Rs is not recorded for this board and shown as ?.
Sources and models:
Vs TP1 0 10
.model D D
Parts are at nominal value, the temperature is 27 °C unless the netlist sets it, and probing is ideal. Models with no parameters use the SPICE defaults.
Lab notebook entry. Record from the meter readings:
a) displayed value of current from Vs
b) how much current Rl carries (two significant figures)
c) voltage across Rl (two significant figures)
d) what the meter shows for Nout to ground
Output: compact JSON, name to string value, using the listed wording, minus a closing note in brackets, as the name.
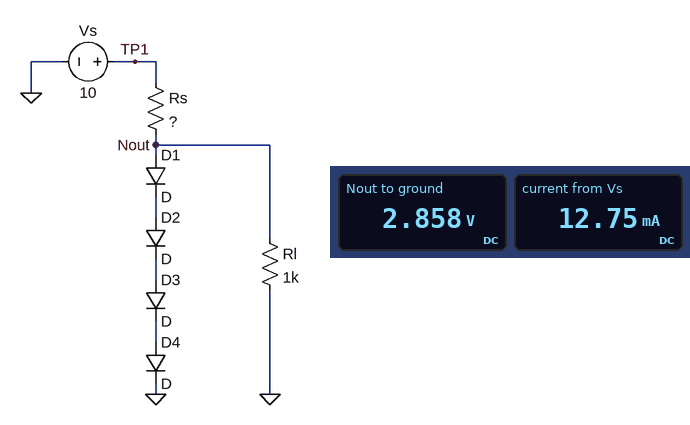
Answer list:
{"displayed value of current from Vs": "12.75 mA", "how much current Rl carries": "2.9 mA", "voltage across Rl": "2.9 V", "what the meter shows for Nout to ground": "2.858 V"}
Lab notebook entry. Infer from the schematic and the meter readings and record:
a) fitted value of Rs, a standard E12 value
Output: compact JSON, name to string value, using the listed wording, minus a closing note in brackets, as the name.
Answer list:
{"fitted value of Rs, a standard E12 value": "560 Ω"}
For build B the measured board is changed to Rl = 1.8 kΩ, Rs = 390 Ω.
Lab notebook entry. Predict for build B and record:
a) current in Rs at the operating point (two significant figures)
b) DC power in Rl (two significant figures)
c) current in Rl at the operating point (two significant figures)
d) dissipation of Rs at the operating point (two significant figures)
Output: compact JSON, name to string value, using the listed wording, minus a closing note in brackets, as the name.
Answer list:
{"current in Rs at the operating point": "18 mA", "DC power in Rl": "4.7 mW", "current in Rl at the operating point": "1.6 mA", "dissipation of Rs at the operating point": "130 mW"}
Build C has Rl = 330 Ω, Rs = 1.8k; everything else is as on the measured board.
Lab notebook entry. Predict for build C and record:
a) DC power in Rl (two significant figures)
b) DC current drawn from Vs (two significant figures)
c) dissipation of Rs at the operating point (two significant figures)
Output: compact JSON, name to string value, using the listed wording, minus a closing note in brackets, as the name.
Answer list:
{"DC power in Rl": "7.3 mW", "DC current drawn from Vs": "4.7 mA", "dissipation of Rs at the operating point": "40 mW"}
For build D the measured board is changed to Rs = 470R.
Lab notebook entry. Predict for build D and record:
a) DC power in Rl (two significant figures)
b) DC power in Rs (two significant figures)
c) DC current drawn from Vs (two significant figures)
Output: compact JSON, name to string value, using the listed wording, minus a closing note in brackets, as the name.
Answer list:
{"DC power in Rl": "8.3 mW", "DC power in Rs": "110 mW", "DC current drawn from Vs": "15 mA"}
